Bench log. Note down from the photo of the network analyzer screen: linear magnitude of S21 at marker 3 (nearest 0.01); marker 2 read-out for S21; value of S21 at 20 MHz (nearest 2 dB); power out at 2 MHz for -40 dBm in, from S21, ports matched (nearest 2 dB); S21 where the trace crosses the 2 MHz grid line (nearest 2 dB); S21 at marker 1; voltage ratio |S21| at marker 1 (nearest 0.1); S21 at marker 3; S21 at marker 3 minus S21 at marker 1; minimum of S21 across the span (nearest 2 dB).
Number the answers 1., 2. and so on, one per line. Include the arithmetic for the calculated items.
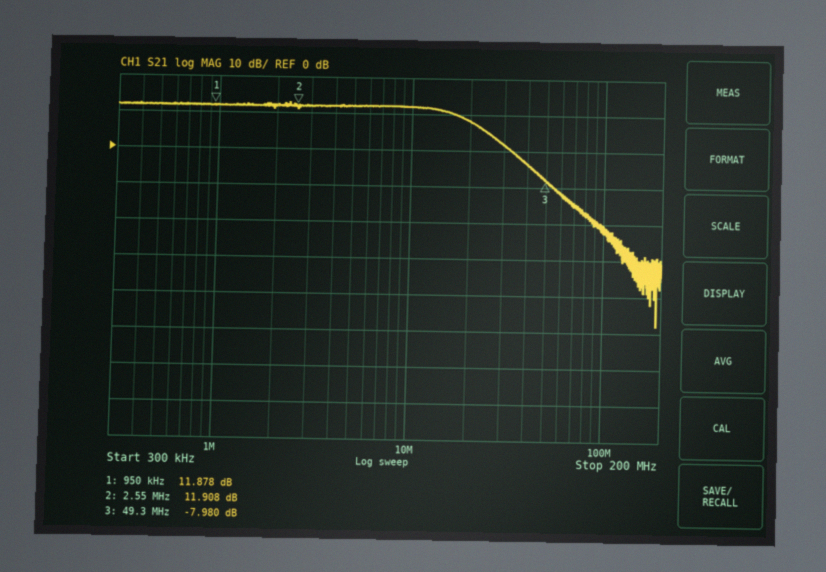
1. 10^(-7.98/20) ≈ 0.40
2. 11.908 dB
3. 8 dB
4. -40 dBm + (12 dB) = -28 dBm
5. 12 dB
6. 11.878 dB
7. 10^(11.878/20) ≈ 3.9
8. -7.980 dB
9. -7.98 − (11.878) = -19.858 dB
10. -48 dB
